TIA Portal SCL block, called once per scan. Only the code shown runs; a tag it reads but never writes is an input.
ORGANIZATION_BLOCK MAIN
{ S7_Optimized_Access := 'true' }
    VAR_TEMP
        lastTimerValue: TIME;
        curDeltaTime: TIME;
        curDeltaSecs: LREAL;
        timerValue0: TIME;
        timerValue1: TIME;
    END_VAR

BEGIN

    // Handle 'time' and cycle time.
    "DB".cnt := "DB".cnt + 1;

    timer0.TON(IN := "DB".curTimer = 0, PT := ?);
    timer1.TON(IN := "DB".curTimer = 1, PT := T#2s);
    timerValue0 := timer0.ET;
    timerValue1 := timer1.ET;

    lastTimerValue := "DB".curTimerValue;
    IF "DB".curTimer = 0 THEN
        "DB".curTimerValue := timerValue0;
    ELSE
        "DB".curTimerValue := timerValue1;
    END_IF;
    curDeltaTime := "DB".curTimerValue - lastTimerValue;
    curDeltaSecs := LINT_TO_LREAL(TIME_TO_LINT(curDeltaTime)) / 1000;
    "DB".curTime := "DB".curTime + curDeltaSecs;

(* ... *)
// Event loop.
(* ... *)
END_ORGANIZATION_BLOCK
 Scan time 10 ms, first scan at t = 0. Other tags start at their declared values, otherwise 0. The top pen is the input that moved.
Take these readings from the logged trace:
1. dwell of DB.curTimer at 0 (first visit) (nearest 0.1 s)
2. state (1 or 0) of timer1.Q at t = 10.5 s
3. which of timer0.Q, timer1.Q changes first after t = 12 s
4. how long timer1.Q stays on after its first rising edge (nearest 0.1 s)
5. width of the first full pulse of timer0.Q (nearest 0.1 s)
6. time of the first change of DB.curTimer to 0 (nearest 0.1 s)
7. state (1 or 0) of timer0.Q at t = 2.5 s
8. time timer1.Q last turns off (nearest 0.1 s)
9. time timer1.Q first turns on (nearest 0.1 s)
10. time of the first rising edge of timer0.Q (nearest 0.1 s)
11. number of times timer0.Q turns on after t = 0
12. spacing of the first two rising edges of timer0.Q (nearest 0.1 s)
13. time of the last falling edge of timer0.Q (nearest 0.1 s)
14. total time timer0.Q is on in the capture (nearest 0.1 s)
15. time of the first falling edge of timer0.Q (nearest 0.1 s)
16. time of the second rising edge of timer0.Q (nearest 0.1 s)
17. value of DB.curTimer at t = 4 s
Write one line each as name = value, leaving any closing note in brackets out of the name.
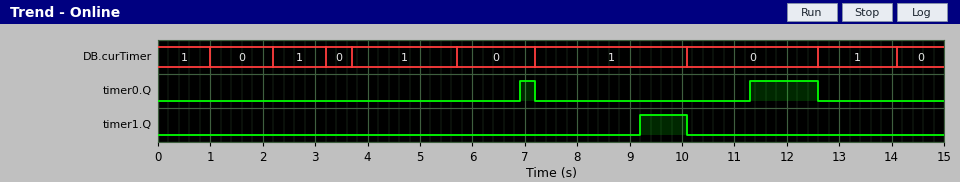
dwell of DB.curTimer at 0 (first visit) = 1.2 s
state (1 or 0) of timer1.Q at t = 10.5 s = 0
which of timer0.Q, timer1.Q changes first after t = 12 s = timer0.Q
how long timer1.Q stays on after its first rising edge = 0.9 s
width of the first full pulse of timer0.Q = 0.3 s
time of the first change of DB.curTimer to 0 = 1.0 s
state (1 or 0) of timer0.Q at t = 2.5 s = 0
time timer1.Q last turns off = 10.1 s
time timer1.Q first turns on = 9.2 s
time of the first rising edge of timer0.Q = 6.9 s
number of times timer0.Q turns on after t = 0 = 2
spacing of the first two rising edges of timer0.Q = 4.4 s
time of the last falling edge of timer0.Q = 12.6 s
total time timer0.Q is on in the capture = 1.6 s
time of the first falling edge of timer0.Q = 7.2 s
time of the second rising edge of timer0.Q = 11.3 s
value of DB.curTimer at t = 4 s = 1
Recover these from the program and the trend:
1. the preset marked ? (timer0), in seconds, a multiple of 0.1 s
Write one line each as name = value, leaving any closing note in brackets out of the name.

the preset marked ? (timer0), in seconds, a multiple of 0.1 s = 1.2 s
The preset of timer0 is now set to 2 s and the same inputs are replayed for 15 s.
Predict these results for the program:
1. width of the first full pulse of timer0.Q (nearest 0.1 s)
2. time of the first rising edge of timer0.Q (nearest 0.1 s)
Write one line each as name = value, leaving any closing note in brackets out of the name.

width of the first full pulse of timer0.Q = 0.5 s
time of the first rising edge of timer0.Q = 12.1 s
